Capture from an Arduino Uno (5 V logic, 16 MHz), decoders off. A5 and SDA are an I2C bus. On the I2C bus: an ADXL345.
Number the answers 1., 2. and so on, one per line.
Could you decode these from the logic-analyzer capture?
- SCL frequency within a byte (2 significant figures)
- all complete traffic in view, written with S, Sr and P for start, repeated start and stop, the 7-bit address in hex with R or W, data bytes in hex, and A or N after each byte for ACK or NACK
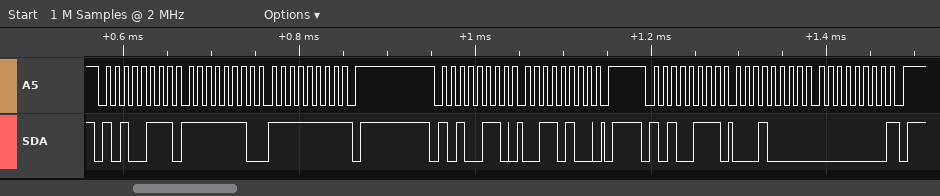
1. 100 kHz
2. S 53R A FE A FF N P S 53W A 34 A P S 53R A 10 A 00 N P
